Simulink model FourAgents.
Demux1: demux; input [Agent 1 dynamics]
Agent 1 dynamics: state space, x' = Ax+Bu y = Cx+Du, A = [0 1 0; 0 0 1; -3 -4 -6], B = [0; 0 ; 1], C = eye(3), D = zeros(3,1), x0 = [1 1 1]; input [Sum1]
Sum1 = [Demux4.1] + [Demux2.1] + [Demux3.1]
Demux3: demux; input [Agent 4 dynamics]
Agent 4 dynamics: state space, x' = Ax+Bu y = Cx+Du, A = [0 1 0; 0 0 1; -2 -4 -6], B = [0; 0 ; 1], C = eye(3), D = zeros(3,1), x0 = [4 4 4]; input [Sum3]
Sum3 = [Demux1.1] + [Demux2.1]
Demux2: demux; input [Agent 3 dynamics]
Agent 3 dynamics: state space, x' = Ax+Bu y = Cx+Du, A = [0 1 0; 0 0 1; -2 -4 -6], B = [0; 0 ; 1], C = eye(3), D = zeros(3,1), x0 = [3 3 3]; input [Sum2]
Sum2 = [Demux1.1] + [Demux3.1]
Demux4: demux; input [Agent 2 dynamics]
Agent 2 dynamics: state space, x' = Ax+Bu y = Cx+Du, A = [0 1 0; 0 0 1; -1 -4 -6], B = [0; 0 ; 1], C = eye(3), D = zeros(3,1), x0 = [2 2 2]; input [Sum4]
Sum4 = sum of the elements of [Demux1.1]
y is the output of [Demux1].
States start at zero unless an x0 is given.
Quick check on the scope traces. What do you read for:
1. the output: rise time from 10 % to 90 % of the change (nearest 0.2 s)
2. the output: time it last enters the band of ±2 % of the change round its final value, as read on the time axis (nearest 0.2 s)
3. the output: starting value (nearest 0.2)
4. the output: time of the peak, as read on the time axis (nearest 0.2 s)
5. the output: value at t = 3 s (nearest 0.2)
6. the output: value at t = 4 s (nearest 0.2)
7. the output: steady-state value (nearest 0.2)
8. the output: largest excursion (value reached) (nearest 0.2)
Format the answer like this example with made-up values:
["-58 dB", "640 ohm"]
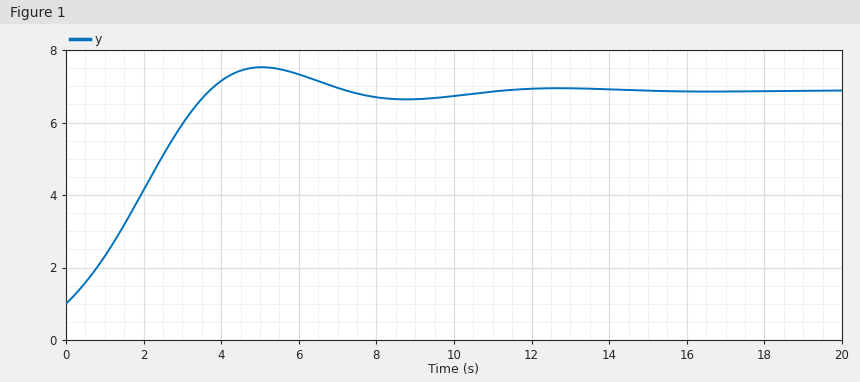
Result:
["2.8 s", "10.2 s", "1.0", "5.0 s", "6.0", "7.2", "6.8", "7.6"]
